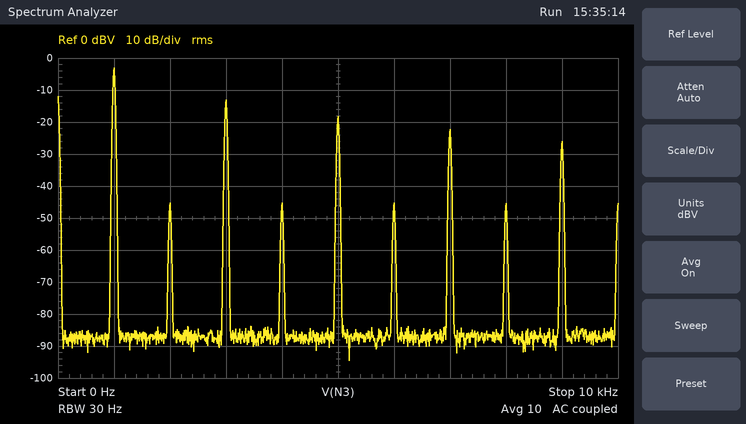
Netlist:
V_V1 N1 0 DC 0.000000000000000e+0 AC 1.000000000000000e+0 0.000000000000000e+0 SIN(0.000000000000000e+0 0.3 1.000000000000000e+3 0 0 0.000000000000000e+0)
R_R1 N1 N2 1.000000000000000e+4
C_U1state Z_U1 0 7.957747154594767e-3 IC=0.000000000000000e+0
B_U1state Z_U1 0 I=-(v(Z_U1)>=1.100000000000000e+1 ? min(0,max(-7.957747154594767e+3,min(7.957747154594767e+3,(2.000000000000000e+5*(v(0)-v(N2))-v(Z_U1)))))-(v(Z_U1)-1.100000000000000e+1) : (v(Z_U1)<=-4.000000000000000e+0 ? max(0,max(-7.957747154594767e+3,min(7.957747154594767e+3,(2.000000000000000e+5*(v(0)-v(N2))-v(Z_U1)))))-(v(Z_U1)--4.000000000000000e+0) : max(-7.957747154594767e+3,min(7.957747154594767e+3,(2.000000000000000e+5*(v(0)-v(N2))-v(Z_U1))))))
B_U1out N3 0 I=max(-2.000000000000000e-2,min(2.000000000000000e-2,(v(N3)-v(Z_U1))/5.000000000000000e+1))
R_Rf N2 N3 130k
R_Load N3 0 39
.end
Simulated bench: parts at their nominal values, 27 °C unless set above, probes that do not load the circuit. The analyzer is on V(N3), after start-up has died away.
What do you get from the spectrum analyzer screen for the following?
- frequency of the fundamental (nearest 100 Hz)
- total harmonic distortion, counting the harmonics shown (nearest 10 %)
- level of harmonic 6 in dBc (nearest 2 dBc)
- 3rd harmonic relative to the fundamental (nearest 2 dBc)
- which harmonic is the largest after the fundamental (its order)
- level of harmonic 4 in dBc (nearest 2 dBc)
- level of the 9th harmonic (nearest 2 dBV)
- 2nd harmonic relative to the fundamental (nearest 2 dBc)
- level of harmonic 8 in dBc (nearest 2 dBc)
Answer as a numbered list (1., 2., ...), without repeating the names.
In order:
1. 1.0 kHz
2. 40 %
3. -42 dBc
4. -10 dBc
5. 3
6. -42 dBc
7. -26 dBV
8. -42 dBc
9. -42 dBc
